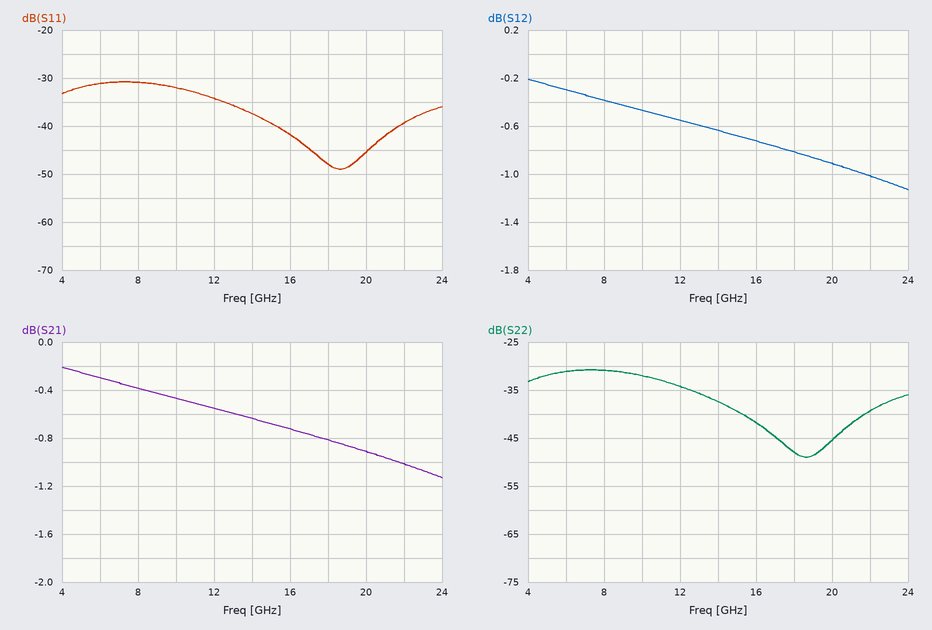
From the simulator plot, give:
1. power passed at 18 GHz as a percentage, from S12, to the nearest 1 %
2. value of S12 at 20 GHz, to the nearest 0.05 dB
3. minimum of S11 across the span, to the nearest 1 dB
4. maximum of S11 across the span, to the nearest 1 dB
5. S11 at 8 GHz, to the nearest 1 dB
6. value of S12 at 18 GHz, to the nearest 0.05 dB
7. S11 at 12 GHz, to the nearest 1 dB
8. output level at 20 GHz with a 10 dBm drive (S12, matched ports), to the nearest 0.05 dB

83 %
-0.90 dB
-49 dB
-31 dB
-31 dB
-0.80 dB
-34 dB
9.10 dBm
